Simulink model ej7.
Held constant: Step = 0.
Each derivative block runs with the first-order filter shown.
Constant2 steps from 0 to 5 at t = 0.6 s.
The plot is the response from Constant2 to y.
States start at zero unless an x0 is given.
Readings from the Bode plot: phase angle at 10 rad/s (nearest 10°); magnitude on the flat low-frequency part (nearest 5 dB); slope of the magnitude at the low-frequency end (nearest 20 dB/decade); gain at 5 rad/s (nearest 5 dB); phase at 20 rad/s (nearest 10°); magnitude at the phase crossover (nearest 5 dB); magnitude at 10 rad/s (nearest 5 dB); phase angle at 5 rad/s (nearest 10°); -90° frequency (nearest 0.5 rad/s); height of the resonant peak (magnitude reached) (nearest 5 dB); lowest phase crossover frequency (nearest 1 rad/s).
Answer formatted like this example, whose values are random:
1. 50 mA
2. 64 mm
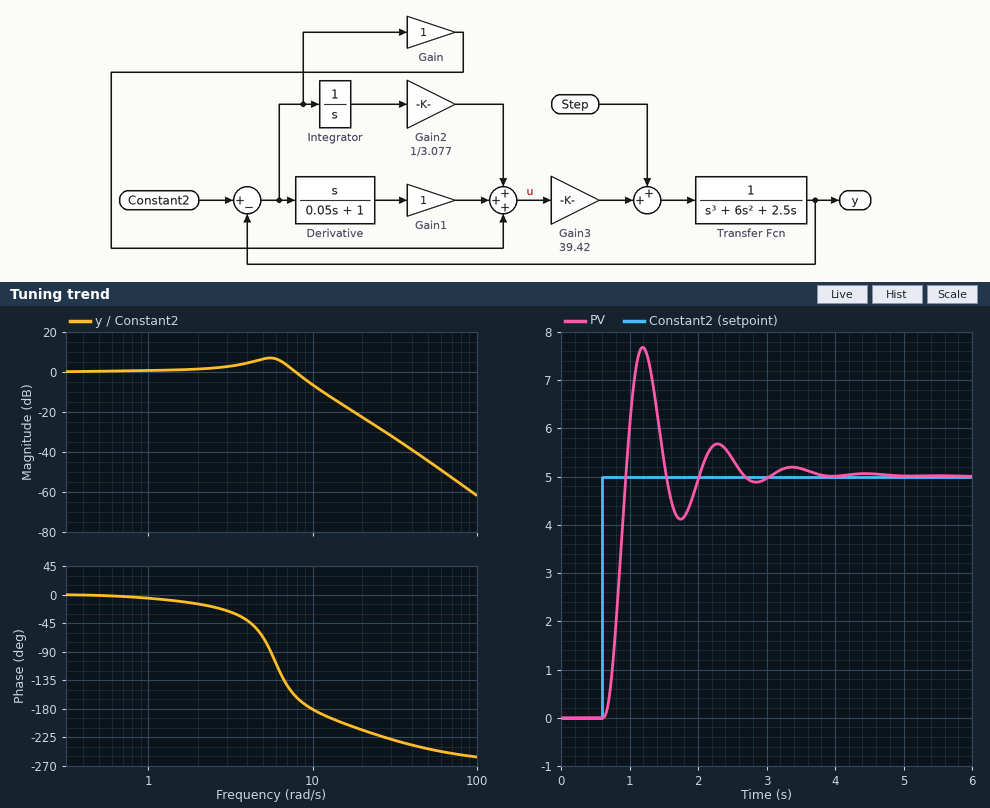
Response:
1. -180°
2. 0 dB
3. 0 dB/decade
4. 5 dB
5. -210°
6. -5 dB
7. -5 dB
8. -70°
9. 5.5 rad/s
10. 5 dB
11. 10 rad/s
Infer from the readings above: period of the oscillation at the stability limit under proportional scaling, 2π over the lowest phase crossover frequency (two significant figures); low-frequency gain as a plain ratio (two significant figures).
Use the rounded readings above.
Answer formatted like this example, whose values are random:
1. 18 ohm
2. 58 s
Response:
1. 0.63 s
2. 1.0
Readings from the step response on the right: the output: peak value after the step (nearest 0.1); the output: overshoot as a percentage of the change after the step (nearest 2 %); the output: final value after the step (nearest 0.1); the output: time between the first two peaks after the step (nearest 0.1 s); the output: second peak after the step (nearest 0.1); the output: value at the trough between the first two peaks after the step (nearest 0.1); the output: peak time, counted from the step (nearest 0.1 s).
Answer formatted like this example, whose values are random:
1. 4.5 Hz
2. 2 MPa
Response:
1. 7.7
2. 54 %
3. 5.0
4. 1.1 s
5. 5.7
6. 4.1
7. 0.6 s
